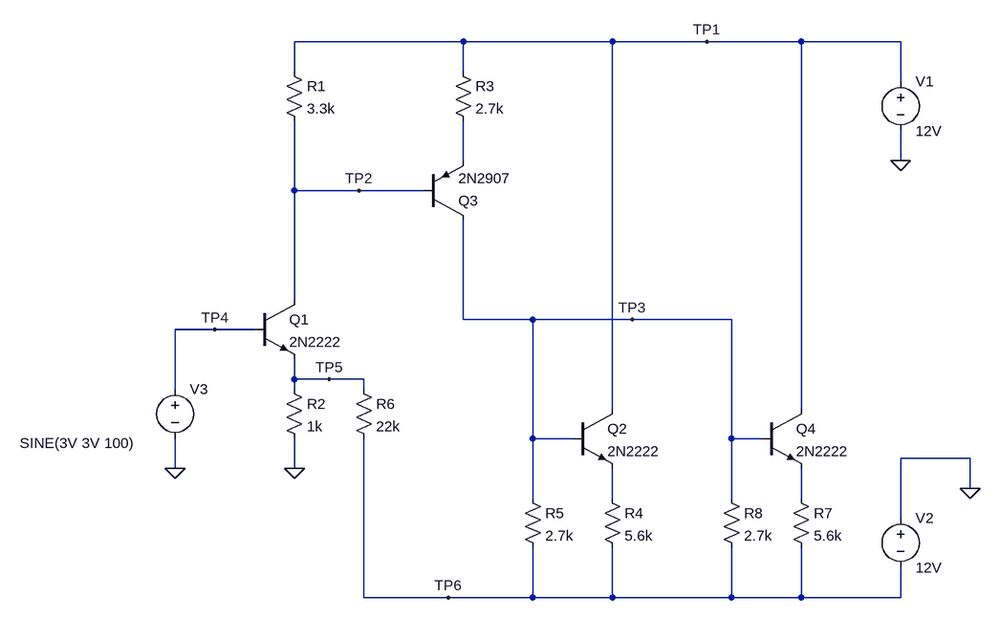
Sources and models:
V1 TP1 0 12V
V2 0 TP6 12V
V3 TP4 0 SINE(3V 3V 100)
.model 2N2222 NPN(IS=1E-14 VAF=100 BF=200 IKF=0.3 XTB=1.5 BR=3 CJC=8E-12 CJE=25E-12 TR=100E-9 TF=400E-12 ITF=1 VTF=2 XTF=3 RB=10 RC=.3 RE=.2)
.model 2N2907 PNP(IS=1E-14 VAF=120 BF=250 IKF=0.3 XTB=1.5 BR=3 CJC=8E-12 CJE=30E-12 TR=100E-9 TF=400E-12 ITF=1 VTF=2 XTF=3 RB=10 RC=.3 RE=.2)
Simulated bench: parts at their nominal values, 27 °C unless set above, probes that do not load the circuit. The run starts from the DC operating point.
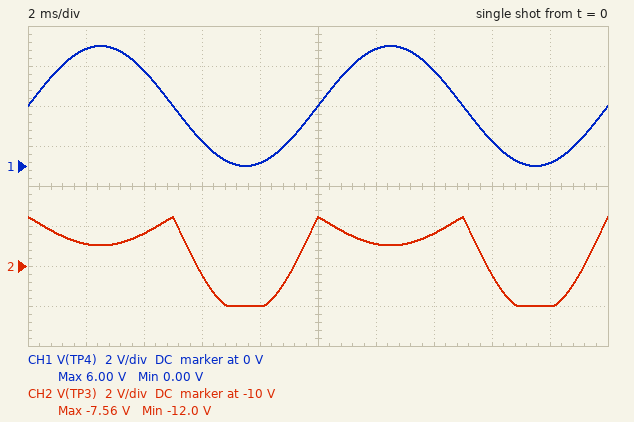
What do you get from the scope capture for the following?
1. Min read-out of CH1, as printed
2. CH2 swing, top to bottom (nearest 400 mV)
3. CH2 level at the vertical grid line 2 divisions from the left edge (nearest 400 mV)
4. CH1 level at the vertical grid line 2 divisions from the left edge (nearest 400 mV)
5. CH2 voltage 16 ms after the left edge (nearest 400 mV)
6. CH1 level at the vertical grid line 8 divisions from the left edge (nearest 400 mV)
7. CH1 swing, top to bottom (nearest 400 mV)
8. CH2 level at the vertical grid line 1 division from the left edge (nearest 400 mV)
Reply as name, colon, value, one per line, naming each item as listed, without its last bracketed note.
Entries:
Min read-out of CH1, as printed: 0.00 V
CH2 swing, top to bottom: 4.4 V
CH2 level at the vertical grid line 2 divisions from the left edge: -8.4 V
CH1 level at the vertical grid line 2 divisions from the left edge: 4.8 V
CH2 voltage 16 ms after the left edge: -10.4 V
CH1 level at the vertical grid line 8 divisions from the left edge: 1.2 V
CH1 swing, top to bottom: 6.0 V
CH2 level at the vertical grid line 1 division from the left edge: -8.8 V
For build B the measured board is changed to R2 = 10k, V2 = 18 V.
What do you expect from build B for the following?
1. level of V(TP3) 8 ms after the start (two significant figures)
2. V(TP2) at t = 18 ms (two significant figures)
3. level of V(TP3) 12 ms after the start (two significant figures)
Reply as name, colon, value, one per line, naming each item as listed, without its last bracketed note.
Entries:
level of V(TP3) 8 ms after the start: -17 V
V(TP2) at t = 18 ms: 9.6 V
level of V(TP3) 12 ms after the start: -16 V
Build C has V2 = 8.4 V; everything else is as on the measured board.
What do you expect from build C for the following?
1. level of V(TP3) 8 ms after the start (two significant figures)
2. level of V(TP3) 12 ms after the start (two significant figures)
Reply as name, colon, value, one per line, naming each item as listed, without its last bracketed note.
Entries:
level of V(TP3) 8 ms after the start: -8.4 V
level of V(TP3) 12 ms after the start: -5.3 V
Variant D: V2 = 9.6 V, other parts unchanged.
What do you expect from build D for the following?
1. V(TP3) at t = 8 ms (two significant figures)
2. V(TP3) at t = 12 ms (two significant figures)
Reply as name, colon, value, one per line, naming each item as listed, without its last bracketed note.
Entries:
V(TP3) at t = 8 ms: -9.6 V
V(TP3) at t = 12 ms: -6.5 V
